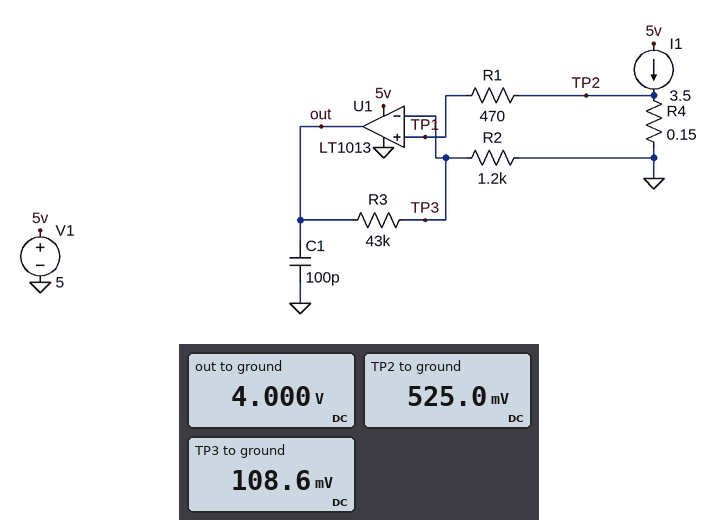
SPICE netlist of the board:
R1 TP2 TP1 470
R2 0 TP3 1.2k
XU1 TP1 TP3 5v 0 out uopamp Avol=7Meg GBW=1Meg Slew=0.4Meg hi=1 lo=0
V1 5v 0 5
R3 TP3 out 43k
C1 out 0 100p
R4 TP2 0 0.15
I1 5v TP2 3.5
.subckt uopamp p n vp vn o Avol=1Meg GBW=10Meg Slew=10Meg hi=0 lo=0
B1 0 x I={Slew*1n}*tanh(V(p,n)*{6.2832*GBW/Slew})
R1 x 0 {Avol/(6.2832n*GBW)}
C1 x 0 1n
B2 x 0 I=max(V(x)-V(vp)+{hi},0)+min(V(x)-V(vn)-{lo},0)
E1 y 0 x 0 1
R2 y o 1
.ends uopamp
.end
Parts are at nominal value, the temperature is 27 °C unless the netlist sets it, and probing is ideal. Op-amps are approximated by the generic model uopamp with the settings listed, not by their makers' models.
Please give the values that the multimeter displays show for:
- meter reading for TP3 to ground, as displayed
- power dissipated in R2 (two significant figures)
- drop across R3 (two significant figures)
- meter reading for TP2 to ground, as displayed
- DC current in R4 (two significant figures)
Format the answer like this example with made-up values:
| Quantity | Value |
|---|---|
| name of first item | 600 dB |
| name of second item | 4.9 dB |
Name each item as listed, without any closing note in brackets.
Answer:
| Quantity | Value |
|---|---|
| meter reading for TP3 to ground, as displayed | 108.6 mV |
| power dissipated in R2 | 9.8 µW |
| drop across R3 | 3.9 V |
| meter reading for TP2 to ground, as displayed | 525.0 mV |
| DC current in R4 | 3.5 A |
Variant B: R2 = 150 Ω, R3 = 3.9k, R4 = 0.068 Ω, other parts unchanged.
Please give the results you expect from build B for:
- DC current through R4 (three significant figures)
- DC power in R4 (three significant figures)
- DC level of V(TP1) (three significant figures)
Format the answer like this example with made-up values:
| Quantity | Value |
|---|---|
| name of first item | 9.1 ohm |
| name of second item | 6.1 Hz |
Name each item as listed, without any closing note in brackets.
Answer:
| Quantity | Value |
|---|---|
| DC current through R4 | 3.50 A |
| DC power in R4 | 833 mW |
| DC level of V(TP1) | 238 mV |
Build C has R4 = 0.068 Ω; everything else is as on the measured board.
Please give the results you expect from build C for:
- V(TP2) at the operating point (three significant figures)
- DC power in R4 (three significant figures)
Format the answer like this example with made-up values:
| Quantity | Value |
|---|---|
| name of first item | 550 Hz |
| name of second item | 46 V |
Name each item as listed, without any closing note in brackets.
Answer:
| Quantity | Value |
|---|---|
| V(TP2) at the operating point | 238 mV |
| DC power in R4 | 833 mW |
